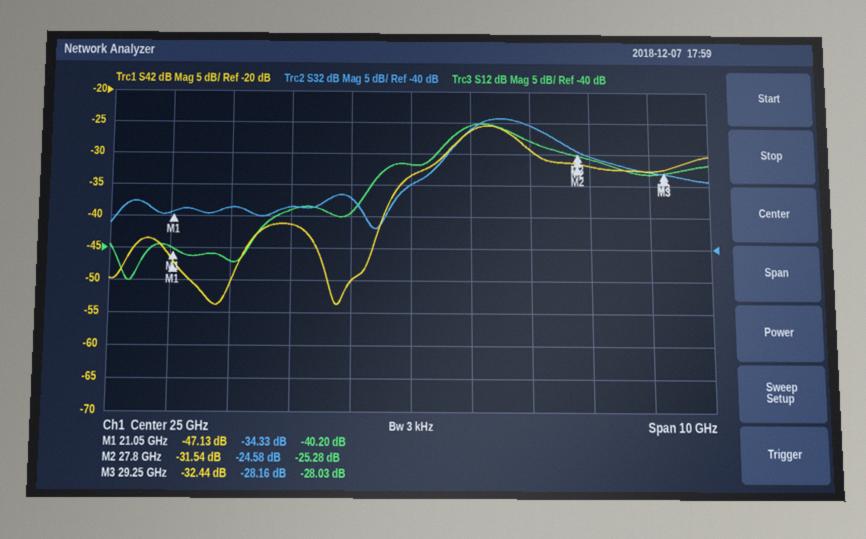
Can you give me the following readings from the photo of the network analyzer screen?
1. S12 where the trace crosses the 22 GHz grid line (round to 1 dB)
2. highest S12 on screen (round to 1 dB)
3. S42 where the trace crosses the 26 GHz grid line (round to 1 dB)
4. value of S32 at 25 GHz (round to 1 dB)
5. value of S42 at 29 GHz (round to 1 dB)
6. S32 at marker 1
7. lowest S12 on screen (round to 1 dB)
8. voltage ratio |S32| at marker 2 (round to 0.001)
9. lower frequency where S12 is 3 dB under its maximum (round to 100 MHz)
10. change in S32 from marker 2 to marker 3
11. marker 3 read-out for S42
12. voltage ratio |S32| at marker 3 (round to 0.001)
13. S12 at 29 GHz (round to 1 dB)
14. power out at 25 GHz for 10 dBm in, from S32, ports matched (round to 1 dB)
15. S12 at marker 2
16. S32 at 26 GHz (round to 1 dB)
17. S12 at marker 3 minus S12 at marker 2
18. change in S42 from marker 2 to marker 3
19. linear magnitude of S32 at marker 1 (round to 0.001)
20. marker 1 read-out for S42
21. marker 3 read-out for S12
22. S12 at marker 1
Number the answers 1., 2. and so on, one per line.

1. -42 dB
2. -20 dB
3. -26 dB
4. -30 dB
5. -33 dB
6. -34.33 dB
7. -45 dB
8. 0.059
9. 25.6 GHz
10. -3.58 dB
11. -32.44 dB
12. 0.039
13. -28 dB
14. -20 dBm
15. -25.28 dB
16. -21 dB
17. -2.75 dB
18. -0.90 dB
19. 0.019
20. -47.13 dB
21. -28.03 dB
22. -40.20 dB
